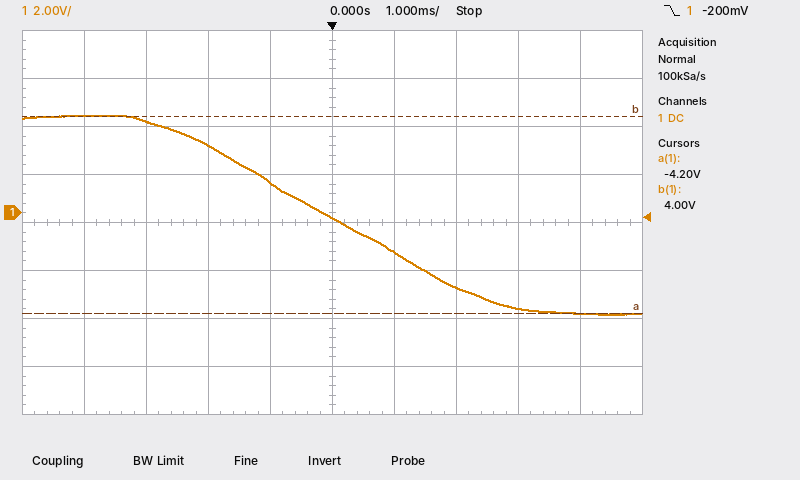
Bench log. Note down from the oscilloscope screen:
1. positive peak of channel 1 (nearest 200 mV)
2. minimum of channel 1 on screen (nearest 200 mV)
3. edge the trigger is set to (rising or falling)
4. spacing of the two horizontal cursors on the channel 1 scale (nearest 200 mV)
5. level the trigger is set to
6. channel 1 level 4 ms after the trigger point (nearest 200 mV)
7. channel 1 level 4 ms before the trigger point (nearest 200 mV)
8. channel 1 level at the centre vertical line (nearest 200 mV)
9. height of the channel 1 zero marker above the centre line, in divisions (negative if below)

4.0 V
-4.2 V
falling
8.2 V
-200 mV
-4.2 V
4.0 V
-200 mV
+0.2 div
